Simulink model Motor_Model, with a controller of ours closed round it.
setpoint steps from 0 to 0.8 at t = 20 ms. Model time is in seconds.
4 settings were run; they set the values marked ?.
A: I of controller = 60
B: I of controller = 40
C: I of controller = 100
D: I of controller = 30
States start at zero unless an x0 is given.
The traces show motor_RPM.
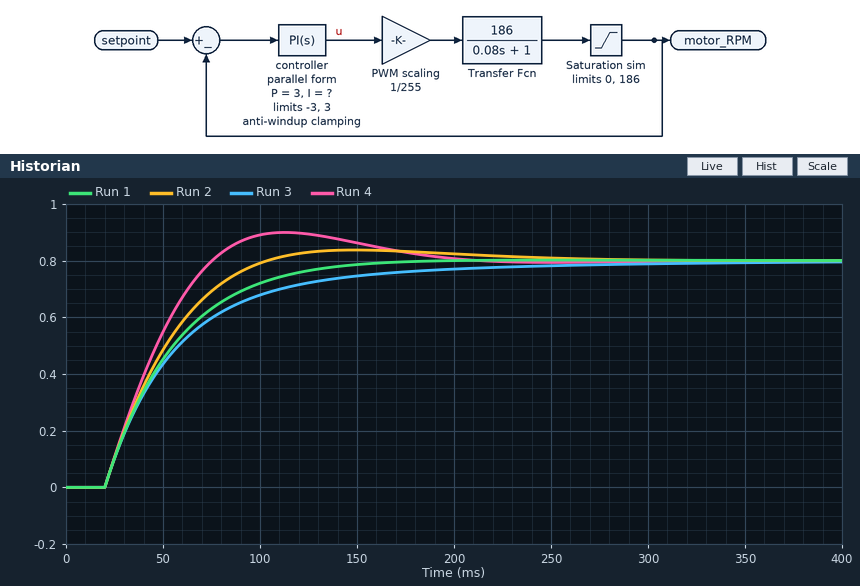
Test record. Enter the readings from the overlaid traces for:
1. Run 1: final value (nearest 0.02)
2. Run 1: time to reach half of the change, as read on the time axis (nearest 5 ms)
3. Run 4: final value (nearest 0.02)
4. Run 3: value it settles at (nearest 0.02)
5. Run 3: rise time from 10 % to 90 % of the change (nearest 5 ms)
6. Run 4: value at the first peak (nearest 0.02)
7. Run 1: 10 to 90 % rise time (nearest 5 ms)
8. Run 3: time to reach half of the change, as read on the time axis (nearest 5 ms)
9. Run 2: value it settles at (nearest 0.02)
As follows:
0.80
45 ms
0.80
0.80
100 ms
0.90
75 ms
45 ms
0.80
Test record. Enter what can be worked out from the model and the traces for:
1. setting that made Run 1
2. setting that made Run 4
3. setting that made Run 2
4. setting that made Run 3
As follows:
B
C
A
D
